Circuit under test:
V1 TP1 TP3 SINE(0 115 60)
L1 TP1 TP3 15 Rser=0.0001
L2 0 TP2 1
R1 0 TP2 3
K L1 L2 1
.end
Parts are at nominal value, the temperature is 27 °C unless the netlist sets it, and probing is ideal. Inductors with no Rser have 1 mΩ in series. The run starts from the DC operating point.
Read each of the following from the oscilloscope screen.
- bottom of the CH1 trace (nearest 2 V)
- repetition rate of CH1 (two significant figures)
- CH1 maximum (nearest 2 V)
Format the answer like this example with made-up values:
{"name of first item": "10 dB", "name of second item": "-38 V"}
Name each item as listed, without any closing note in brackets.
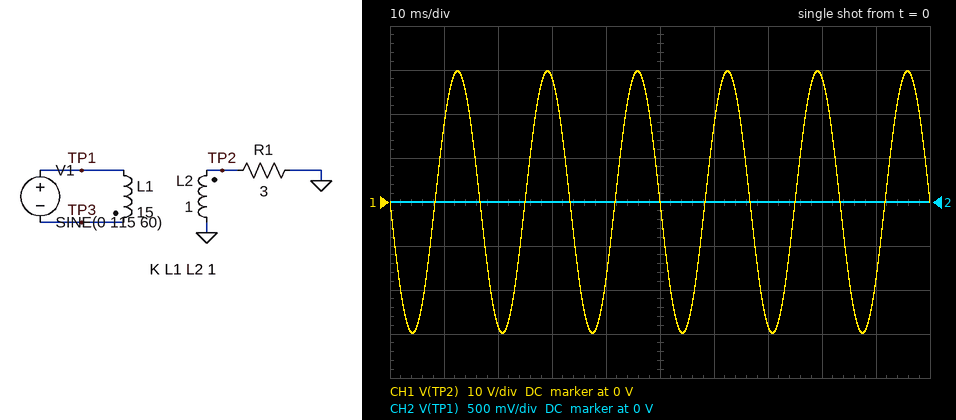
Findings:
{"bottom of the CH1 trace": "-30 V", "repetition rate of CH1": "60 Hz", "CH1 maximum": "30 V"}
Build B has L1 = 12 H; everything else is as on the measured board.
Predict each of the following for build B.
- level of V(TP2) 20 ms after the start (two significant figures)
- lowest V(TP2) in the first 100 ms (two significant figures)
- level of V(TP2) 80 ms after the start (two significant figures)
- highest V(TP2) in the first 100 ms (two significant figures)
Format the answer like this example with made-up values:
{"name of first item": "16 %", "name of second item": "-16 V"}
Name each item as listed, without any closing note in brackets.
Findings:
{"level of V(TP2) 20 ms after the start": "-32 V", "lowest V(TP2) in the first 100 ms": "-33 V", "level of V(TP2) 80 ms after the start": "32 V", "highest V(TP2) in the first 100 ms": "33 V"}
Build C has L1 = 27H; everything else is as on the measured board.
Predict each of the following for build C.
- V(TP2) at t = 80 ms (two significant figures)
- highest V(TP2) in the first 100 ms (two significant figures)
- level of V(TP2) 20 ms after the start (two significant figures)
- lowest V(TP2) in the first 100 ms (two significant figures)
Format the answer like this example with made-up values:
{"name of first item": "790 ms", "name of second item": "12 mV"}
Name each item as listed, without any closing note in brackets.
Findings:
{"V(TP2) at t = 80 ms": "21 V", "highest V(TP2) in the first 100 ms": "22 V", "level of V(TP2) 20 ms after the start": "-21 V", "lowest V(TP2) in the first 100 ms": "-22 V"}
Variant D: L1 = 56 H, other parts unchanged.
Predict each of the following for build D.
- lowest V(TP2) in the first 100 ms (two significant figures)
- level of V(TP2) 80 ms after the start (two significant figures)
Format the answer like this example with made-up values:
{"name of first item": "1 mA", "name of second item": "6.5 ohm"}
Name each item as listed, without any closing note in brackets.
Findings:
{"lowest V(TP2) in the first 100 ms": "-15 V", "level of V(TP2) 80 ms after the start": "15 V"}
